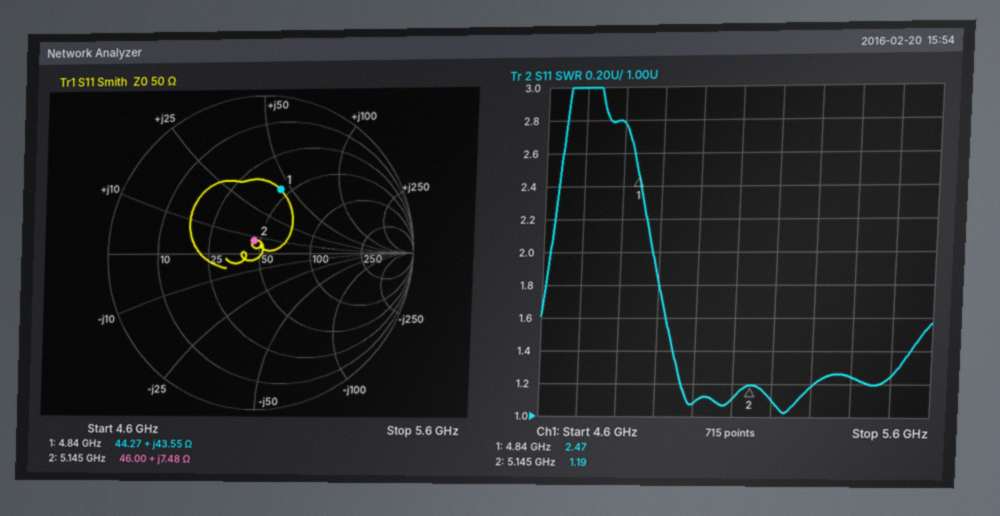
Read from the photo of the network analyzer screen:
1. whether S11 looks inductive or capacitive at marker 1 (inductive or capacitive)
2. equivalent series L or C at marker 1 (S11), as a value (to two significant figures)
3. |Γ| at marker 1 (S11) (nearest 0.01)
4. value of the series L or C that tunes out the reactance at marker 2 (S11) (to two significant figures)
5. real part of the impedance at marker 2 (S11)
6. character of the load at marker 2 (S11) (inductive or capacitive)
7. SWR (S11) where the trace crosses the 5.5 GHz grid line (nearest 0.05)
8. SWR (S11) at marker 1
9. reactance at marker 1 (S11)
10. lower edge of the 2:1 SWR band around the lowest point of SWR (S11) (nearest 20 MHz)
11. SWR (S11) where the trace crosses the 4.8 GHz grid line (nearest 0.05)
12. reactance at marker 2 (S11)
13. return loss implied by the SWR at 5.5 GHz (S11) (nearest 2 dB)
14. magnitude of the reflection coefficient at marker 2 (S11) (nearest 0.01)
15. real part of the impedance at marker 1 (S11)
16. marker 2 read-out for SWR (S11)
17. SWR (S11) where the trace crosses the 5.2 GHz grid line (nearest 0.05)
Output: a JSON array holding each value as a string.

["inductive", "1.4 nH", "0.42", "4.1 pF", "46.00 Ω", "inductive", "1.25", "2.47", "+43.55 Ω", "4.88 GHz", "2.80", "+7.48 Ω", "20 dB", "0.09", "44.27 Ω", "1.19", "1.10"]
